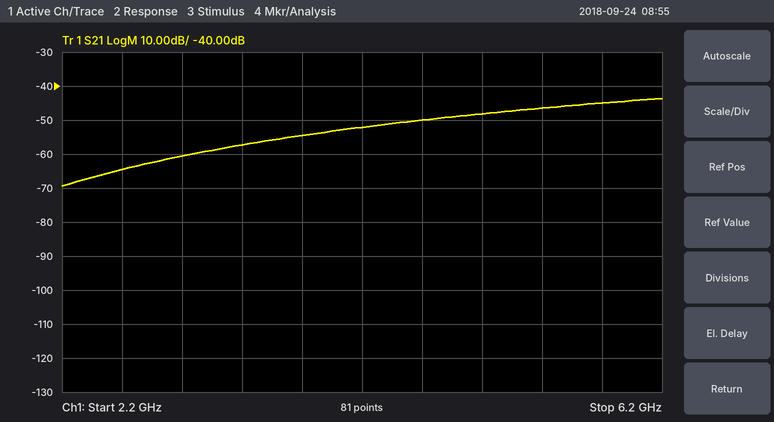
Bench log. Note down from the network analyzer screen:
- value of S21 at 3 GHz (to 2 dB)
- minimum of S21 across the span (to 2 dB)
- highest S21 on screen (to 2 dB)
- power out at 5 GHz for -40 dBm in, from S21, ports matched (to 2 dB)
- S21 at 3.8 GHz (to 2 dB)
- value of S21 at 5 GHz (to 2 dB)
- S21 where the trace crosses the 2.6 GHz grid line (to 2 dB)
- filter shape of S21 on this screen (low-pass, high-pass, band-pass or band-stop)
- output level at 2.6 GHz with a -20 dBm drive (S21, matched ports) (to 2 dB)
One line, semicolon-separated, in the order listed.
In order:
-60 dB; -70 dB; -44 dB; -88 dBm; -54 dB; -48 dB; -64 dB; high-pass; -84 dBm
